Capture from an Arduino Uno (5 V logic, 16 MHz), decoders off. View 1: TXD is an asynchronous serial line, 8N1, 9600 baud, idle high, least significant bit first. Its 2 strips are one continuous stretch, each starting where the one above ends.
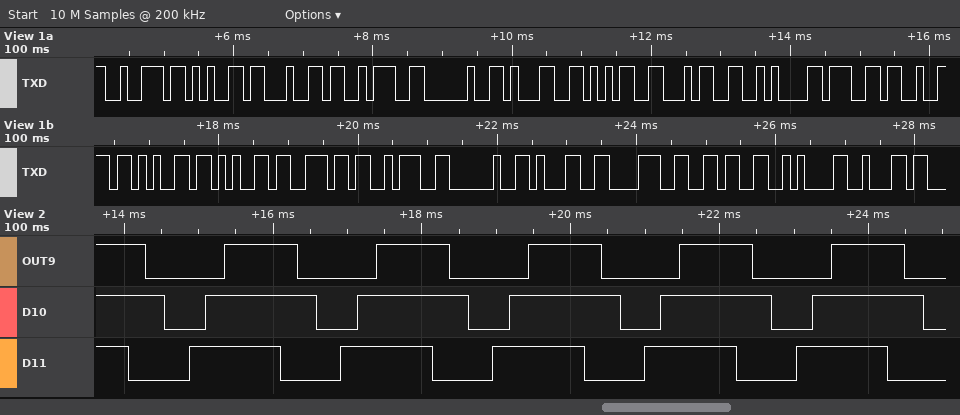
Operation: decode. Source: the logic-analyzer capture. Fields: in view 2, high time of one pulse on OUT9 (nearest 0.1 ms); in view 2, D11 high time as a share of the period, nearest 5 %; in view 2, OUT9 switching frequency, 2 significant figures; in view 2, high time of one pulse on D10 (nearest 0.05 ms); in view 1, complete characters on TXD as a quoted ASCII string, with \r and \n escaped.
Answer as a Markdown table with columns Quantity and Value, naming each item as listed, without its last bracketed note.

| Quantity | Value |
|---|---|
| in view 2, high time of one pulse on OUT9 | 1.0 ms |
| in view 2, D11 high time as a share of the period, nearest 5 % | 60 % |
| in view 2, OUT9 switching frequency, 2 significant figures | 490 Hz |
| in view 2, high time of one pulse on D10 | 1.50 ms |
| in view 1, complete characters on TXD as a quoted ASCII string, with \r and \n escaped | "red: 154\ngreen: 186\nb" |
